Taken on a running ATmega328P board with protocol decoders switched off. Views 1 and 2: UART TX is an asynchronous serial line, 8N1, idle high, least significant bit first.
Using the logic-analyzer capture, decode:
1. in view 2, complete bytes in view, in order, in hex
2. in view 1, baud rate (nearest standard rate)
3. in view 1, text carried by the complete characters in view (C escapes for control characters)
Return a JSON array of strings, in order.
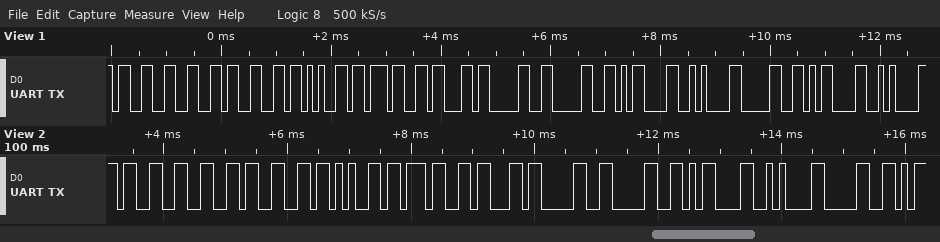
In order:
["0x33 0x66 0x66 0x65 0x37 0x63 0x30 0x30 0x0D 0x0A 0x30", "9600 baud", "\"3ffe7c00\\r\\n0\\r\\n\""]
